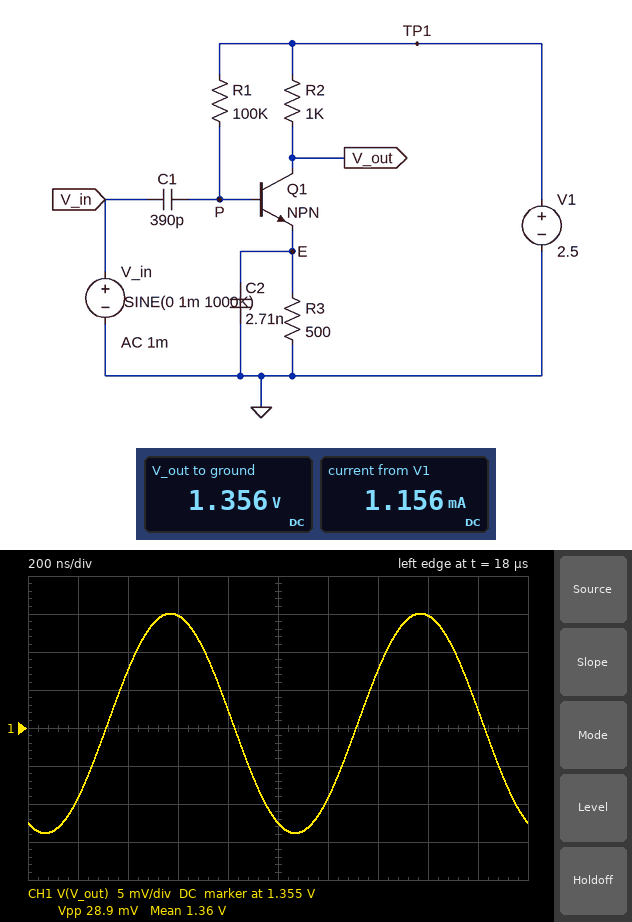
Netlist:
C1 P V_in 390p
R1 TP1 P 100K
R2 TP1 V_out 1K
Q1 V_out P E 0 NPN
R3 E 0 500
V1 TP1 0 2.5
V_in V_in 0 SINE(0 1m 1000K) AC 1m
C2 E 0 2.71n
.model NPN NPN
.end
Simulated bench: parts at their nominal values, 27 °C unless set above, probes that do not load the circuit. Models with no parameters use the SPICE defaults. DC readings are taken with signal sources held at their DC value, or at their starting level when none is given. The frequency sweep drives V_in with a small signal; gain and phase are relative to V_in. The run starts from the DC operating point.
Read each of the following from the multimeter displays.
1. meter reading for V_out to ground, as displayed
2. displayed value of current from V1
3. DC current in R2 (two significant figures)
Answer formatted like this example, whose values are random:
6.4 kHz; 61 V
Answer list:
1.356 V; 1.156 mA; 1.1 mA
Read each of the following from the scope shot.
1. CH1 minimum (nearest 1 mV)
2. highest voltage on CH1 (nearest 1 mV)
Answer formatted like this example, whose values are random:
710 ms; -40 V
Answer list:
1.341 V; 1.370 V
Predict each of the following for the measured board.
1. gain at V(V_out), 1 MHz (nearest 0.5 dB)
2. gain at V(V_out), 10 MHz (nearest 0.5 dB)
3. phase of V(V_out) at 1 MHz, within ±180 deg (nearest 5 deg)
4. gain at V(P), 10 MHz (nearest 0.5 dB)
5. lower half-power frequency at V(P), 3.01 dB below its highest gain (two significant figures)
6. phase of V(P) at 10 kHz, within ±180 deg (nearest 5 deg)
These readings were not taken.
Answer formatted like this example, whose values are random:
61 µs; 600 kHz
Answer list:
23.0 dB; 32.5 dB; -115 deg; 0 dB; 13 kHz; 50 deg
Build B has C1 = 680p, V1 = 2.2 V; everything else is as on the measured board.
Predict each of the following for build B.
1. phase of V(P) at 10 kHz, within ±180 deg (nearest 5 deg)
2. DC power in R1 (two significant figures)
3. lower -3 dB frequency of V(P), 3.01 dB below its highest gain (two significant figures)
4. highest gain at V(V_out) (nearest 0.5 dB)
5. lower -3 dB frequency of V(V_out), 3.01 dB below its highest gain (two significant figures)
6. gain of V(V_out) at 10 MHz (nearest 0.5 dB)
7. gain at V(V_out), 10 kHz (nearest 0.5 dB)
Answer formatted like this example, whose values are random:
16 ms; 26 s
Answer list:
35 deg; 9.0 µW; 7.0 kHz; 31.5 dB; 2.4 MHz; 31.0 dB; 3.5 dB
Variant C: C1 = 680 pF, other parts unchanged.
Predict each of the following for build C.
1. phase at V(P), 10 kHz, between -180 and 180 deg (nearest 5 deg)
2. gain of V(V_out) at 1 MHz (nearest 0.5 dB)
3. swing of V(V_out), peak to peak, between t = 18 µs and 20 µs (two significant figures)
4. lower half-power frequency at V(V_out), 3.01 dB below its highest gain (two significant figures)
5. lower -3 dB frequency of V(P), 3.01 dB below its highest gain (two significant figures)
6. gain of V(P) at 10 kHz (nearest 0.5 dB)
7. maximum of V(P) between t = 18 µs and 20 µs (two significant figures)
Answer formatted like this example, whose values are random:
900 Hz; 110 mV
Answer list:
35 deg; 23.5 dB; 30 mV; 2.8 MHz; 7.0 kHz; -2.0 dB; 1.4 V
